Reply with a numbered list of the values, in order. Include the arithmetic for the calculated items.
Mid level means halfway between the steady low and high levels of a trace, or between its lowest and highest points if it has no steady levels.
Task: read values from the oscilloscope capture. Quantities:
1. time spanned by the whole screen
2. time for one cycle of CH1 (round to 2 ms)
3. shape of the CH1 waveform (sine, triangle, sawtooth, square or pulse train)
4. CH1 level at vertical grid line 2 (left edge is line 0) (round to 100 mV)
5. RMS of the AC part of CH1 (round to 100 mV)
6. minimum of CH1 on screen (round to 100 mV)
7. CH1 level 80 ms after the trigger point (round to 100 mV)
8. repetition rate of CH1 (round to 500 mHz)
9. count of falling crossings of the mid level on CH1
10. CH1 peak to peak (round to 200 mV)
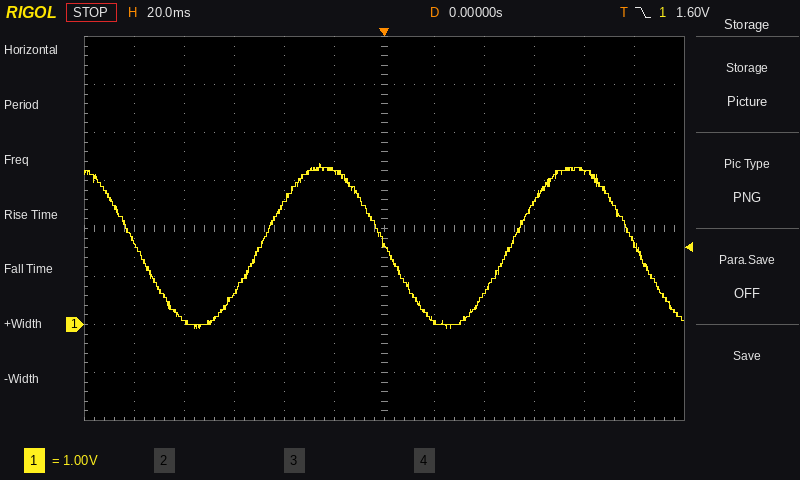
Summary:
1. 240 ms
2. 100 ms
3. sine
4. 100 mV
5. 3.4 V / (2√2) ≈ 1.2 V
6. -100 mV
7. 3.2 V
8. 1 / 100 ms ≈ 10.0 Hz
9. 3
10. 3.4 V
